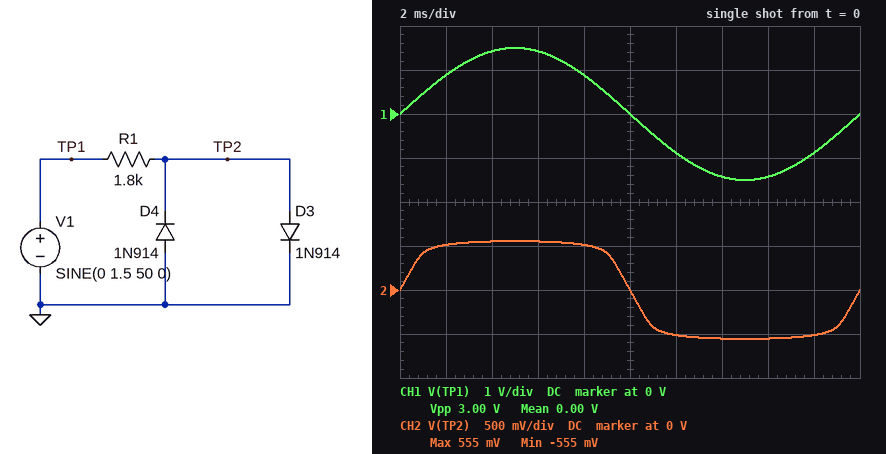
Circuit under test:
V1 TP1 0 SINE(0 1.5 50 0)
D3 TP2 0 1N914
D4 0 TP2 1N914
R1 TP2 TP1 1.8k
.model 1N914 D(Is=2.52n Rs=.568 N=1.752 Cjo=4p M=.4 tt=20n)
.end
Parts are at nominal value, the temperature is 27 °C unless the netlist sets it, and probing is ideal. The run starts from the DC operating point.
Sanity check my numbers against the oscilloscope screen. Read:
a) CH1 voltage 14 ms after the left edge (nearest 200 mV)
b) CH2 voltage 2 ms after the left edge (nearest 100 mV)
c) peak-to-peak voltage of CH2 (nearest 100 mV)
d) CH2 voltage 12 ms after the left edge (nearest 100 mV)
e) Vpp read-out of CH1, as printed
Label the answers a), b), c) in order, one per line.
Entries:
a) -1.4 V
b) 500 mV
c) 1.1 V
d) -500 mV
e) 3.00 V
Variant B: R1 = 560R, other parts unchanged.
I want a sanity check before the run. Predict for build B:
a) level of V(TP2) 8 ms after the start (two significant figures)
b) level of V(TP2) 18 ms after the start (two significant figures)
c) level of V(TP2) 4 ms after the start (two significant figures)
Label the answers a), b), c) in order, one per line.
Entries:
a) 560 mV
b) -560 mV
c) 600 mV
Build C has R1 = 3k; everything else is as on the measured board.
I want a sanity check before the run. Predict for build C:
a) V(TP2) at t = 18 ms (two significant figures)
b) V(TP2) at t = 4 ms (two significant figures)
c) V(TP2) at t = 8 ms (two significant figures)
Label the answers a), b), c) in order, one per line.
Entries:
a) -490 mV
b) 530 mV
c) 490 mV
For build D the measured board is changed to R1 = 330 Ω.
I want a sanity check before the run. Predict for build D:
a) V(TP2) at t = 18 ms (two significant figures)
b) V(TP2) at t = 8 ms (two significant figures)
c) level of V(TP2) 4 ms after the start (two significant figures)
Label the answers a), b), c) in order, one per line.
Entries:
a) -580 mV
b) 580 mV
c) 630 mV
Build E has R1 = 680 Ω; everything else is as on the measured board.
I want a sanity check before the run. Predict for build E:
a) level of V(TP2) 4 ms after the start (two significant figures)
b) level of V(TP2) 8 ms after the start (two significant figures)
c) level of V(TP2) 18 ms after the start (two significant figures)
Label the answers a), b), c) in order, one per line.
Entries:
a) 590 mV
b) 550 mV
c) -550 mV
